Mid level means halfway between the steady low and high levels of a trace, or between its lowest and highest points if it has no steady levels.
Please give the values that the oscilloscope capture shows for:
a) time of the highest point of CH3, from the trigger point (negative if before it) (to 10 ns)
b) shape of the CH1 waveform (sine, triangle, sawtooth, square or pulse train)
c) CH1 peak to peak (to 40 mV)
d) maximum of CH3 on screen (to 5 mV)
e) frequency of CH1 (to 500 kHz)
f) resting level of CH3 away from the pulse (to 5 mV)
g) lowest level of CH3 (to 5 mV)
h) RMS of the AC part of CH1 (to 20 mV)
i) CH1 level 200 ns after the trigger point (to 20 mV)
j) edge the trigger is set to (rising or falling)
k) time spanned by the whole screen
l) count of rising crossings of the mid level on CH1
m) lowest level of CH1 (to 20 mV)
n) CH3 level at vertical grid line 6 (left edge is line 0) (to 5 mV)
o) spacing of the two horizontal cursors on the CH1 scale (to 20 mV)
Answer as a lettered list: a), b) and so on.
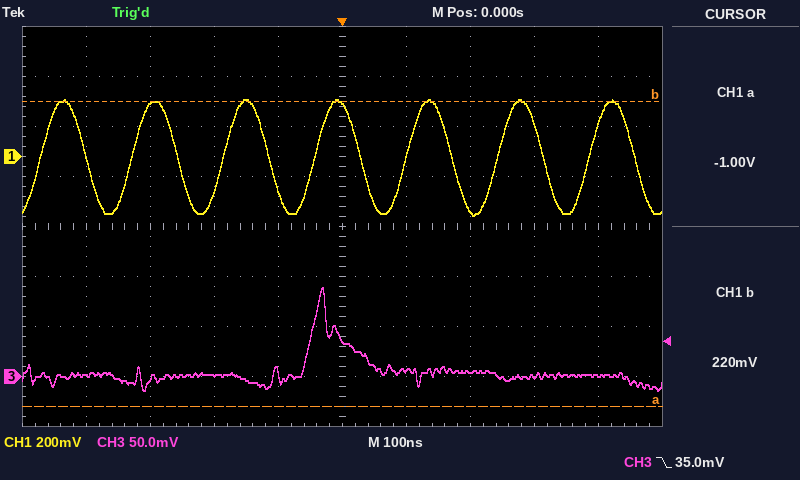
a) -30 ns
b) sine
c) 480 mV
d) 90 mV
e) 7.0 MHz
f) 0 mV
g) -15 mV
h) 160 mV
i) -220 mV
j) falling
k) 1 µs
l) 7
m) -240 mV
n) 5 mV
o) 1.22 V
